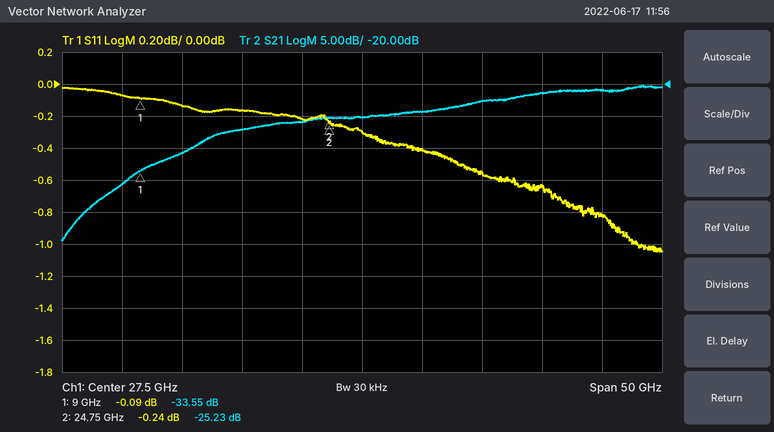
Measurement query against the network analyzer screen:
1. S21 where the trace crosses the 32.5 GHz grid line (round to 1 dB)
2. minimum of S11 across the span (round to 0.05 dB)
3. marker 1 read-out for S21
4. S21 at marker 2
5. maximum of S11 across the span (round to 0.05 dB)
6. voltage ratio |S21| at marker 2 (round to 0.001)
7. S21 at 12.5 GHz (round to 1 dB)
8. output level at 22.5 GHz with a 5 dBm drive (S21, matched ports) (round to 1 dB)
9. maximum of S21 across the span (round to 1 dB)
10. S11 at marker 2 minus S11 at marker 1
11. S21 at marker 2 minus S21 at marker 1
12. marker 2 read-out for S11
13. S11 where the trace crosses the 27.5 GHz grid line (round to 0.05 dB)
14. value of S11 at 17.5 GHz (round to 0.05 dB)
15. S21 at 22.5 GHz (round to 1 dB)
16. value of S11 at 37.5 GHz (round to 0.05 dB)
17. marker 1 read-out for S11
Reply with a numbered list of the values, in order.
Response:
1. -24 dB
2. -1.05 dB
3. -33.55 dB
4. -25.23 dB
5. 0.00 dB
6. 0.055
7. -31 dB
8. -21 dBm
9. -20 dB
10. -0.15 dB
11. 8.32 dB
12. -0.24 dB
13. -0.30 dB
14. -0.15 dB
15. -26 dB
16. -0.55 dB
17. -0.09 dB
